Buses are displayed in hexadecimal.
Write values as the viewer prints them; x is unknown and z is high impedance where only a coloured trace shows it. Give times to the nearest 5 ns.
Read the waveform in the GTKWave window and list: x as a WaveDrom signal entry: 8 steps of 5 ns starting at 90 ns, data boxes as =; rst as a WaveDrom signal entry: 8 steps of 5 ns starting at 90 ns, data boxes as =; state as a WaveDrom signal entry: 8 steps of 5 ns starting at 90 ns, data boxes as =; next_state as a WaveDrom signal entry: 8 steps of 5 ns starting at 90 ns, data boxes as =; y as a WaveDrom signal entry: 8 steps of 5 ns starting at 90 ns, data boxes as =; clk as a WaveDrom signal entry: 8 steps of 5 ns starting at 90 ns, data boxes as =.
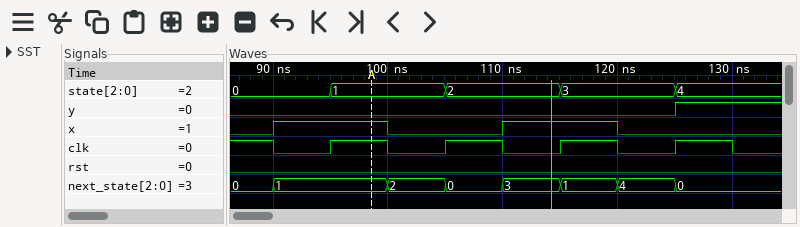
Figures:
{name: 'x', wave: '1.0.1.0.'}
{name: 'rst', wave: '0.......'}
{name: 'state', wave: '==.=.=.=', data: '0 1 2 3 4'}
{name: 'next_state', wave: '=.======', data: '1 2 0 3 1 4 0'}
{name: 'y', wave: '0......1'}
{name: 'clk', wave: '01010101'}
